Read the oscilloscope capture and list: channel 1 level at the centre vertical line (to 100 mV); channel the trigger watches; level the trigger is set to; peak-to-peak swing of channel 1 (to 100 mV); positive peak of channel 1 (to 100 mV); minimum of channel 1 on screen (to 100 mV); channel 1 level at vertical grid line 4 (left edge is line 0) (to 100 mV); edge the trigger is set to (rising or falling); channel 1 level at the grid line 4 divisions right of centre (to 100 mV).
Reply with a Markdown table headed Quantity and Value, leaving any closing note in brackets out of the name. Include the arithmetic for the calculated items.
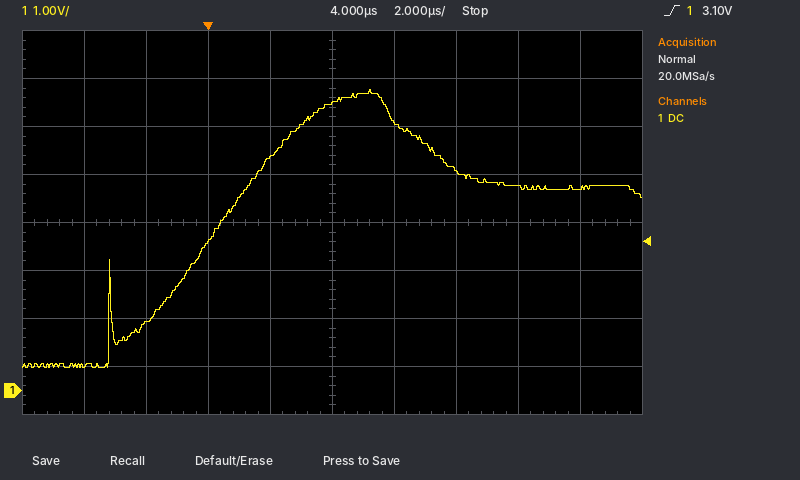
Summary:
| Quantity | Value |
|---|---|
| channel 1 level at the centre vertical line | 6.0 V |
| channel the trigger watches | channel 1 |
| level the trigger is set to | 3.10 V |
| peak-to-peak swing of channel 1 | 6.3 V − (500 mV) = 5.8 V |
| positive peak of channel 1 | 6.3 V |
| minimum of channel 1 on screen | 500 mV |
| channel 1 level at vertical grid line 4 (left edge is line 0) | 4.9 V |
| edge the trigger is set to | rising |
| channel 1 level at the grid line 4 divisions right of centre | 4.2 V |
